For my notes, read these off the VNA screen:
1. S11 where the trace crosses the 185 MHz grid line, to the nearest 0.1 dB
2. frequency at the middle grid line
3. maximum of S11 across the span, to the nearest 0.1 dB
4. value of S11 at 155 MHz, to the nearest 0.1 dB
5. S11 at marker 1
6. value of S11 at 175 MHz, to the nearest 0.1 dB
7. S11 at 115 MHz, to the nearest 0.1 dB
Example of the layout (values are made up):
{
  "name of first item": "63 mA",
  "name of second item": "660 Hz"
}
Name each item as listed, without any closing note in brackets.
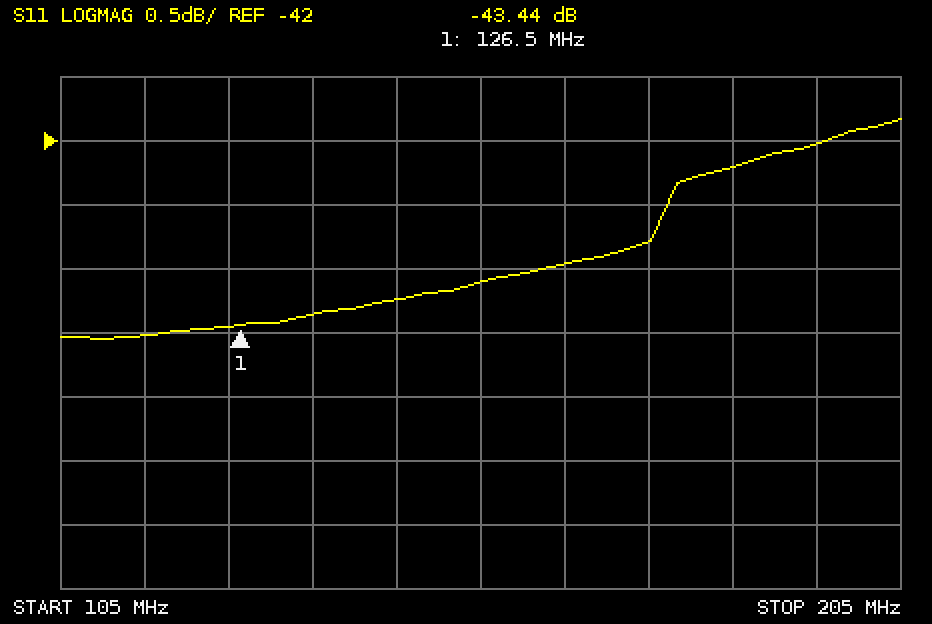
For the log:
{
  "S11 where the trace crosses the 185 MHz grid line, to the nearest 0.1 dB": "-42.2 dB",
  "frequency at the middle grid line": "155 MHz",
  "maximum of S11 across the span, to the nearest 0.1 dB": "-41.8 dB",
  "value of S11 at 155 MHz, to the nearest 0.1 dB": "-43.1 dB",
  "S11 at marker 1": "-43.44 dB",
  "value of S11 at 175 MHz, to the nearest 0.1 dB": "-42.8 dB",
  "S11 at 115 MHz, to the nearest 0.1 dB": "-43.5 dB"
}
